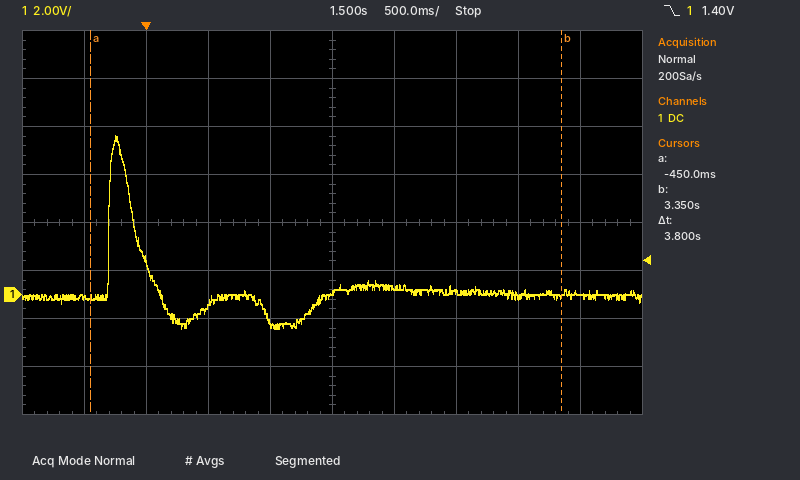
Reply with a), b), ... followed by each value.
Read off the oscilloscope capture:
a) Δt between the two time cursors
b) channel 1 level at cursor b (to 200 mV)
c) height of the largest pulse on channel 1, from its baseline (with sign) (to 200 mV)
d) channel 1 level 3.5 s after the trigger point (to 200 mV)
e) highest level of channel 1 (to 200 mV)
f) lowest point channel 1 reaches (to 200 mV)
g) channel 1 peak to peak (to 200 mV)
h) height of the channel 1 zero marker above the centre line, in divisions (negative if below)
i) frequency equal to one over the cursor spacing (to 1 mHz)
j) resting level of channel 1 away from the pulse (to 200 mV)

a) 3.8 s
b) 0.0 V
c) +6.6 V
d) 0.0 V
e) 6.6 V
f) -1.4 V
g) 8.0 V
h) -1.5 div
i) 263 mHz
j) 0.0 V
